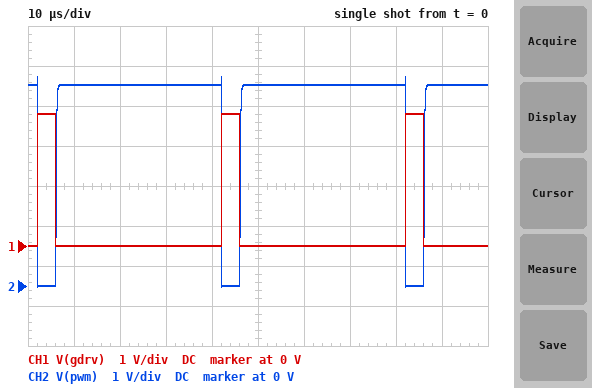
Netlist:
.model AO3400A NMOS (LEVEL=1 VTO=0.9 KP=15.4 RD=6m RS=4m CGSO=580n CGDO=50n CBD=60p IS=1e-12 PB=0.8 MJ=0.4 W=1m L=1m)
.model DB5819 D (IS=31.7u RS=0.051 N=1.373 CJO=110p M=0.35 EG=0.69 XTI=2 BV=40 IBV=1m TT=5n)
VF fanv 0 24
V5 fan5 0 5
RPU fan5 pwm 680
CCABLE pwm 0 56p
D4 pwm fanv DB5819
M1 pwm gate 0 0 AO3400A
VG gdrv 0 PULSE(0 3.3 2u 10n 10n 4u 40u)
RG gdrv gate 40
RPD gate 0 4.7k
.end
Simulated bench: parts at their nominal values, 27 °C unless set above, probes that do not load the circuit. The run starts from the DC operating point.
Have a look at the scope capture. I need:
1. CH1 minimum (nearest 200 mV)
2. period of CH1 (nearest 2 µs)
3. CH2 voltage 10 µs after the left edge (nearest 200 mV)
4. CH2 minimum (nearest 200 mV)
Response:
0 V
40 µs
5.0 V
0 V
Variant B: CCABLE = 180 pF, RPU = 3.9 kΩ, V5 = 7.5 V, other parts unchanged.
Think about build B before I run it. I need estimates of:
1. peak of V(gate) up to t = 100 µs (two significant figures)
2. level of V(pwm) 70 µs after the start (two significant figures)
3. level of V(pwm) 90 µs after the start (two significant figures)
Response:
3.3 V
7.6 V
7.4 V
